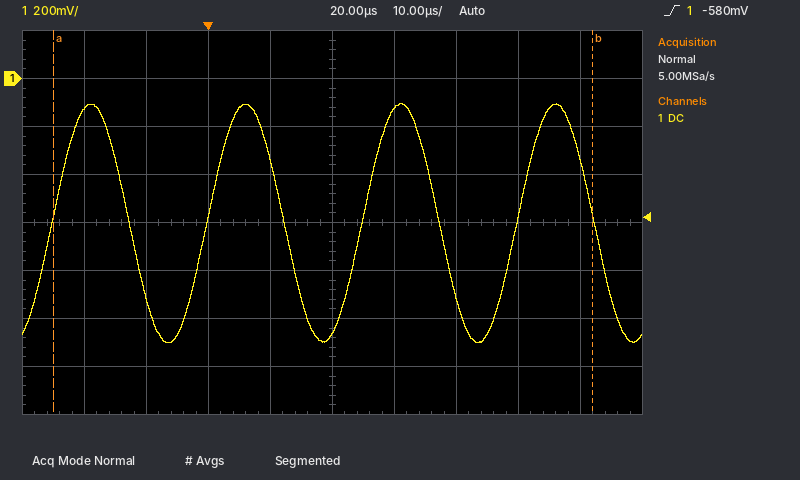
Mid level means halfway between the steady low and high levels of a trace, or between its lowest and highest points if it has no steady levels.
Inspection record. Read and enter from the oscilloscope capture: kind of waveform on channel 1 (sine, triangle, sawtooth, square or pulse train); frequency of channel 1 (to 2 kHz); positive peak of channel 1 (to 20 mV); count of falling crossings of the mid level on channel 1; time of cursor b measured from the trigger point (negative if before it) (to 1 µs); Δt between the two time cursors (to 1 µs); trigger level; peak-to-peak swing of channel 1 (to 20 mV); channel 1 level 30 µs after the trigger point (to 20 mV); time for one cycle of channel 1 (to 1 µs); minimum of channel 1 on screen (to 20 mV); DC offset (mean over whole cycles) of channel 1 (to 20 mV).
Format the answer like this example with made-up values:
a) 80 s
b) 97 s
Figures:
a) sine
b) 40 kHz
c) -100 mV
d) 4
e) +62 µs
f) 87 µs
g) -580 mV
h) 1.00 V
i) -120 mV
j) 25 µs
k) -1.10 V
l) -600 mV
